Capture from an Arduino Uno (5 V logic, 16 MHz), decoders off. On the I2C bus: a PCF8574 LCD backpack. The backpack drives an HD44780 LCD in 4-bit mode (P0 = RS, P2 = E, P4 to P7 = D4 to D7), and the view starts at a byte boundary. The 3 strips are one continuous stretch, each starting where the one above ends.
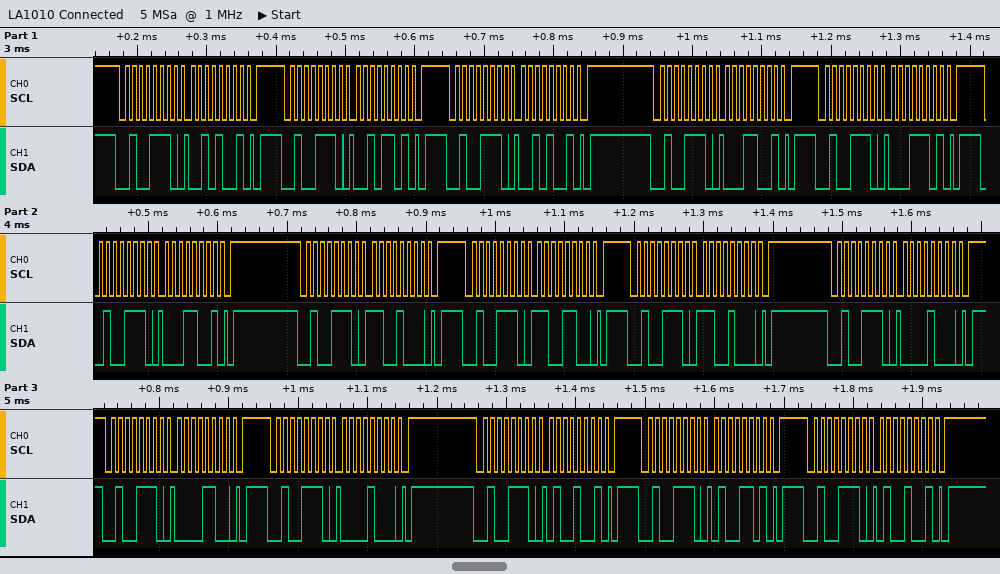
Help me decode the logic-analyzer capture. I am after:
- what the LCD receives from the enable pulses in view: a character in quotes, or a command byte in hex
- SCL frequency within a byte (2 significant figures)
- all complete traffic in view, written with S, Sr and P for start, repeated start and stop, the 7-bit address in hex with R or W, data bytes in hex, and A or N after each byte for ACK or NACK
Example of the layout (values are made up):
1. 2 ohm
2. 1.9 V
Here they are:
1. '!' 0xC0
2. 100 kHz
3. S 27W A 29 A P S 27W A 2D A P S 27W A 29 A P S 27W A 19 A P S 27W A 1D A P S 27W A 19 A P S 27W A C8 A P S 27W A CC A P S 27W A C8 A P S 27W A 08 A P S 27W A 0C A P S 27W A 08 A P S 27W A 49 A P S 27W A 4D A P S 27W A 49 A P
